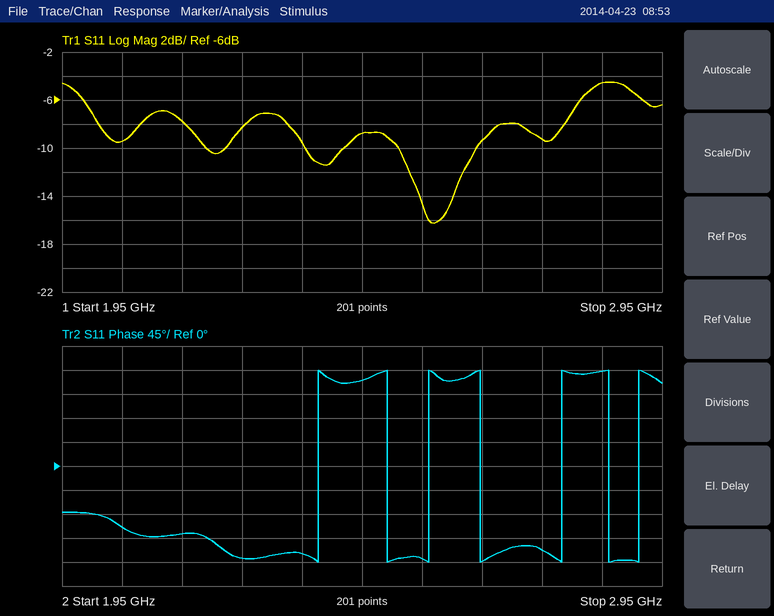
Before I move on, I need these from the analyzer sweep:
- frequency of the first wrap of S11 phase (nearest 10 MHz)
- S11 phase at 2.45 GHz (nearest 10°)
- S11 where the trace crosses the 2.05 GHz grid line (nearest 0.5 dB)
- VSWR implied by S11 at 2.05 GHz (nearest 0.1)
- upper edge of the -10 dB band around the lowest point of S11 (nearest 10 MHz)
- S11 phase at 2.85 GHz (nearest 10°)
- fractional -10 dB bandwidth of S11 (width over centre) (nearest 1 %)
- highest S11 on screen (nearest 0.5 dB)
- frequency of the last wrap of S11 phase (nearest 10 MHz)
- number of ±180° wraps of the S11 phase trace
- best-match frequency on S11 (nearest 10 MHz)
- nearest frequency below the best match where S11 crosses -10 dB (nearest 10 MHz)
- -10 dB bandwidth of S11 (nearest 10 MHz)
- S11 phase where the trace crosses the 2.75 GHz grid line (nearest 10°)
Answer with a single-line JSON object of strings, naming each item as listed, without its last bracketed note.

{"frequency of the first wrap of S11 phase": "2.38 GHz", "S11 phase at 2.45 GHz": "160°", "S11 where the trace crosses the 2.05 GHz grid line": "-9.5 dB", "VSWR implied by S11 at 2.05 GHz": "2.0", "upper edge of the -10 dB band around the lowest point of S11": "2.64 GHz", "S11 phase at 2.85 GHz": "180°", "fractional -10 dB bandwidth of S11 (width over centre)": "5 %", "highest S11 on screen": "-4.5 dB", "frequency of the last wrap of S11 phase": "2.91 GHz", "number of ±180° wraps of the S11 phase trace": "7", "best-match frequency on S11": "2.57 GHz", "nearest frequency below the best match where S11 crosses -10 dB": "2.51 GHz", "-10 dB bandwidth of S11": "130 MHz", "S11 phase where the trace crosses the 2.75 GHz grid line": "-160°"}
